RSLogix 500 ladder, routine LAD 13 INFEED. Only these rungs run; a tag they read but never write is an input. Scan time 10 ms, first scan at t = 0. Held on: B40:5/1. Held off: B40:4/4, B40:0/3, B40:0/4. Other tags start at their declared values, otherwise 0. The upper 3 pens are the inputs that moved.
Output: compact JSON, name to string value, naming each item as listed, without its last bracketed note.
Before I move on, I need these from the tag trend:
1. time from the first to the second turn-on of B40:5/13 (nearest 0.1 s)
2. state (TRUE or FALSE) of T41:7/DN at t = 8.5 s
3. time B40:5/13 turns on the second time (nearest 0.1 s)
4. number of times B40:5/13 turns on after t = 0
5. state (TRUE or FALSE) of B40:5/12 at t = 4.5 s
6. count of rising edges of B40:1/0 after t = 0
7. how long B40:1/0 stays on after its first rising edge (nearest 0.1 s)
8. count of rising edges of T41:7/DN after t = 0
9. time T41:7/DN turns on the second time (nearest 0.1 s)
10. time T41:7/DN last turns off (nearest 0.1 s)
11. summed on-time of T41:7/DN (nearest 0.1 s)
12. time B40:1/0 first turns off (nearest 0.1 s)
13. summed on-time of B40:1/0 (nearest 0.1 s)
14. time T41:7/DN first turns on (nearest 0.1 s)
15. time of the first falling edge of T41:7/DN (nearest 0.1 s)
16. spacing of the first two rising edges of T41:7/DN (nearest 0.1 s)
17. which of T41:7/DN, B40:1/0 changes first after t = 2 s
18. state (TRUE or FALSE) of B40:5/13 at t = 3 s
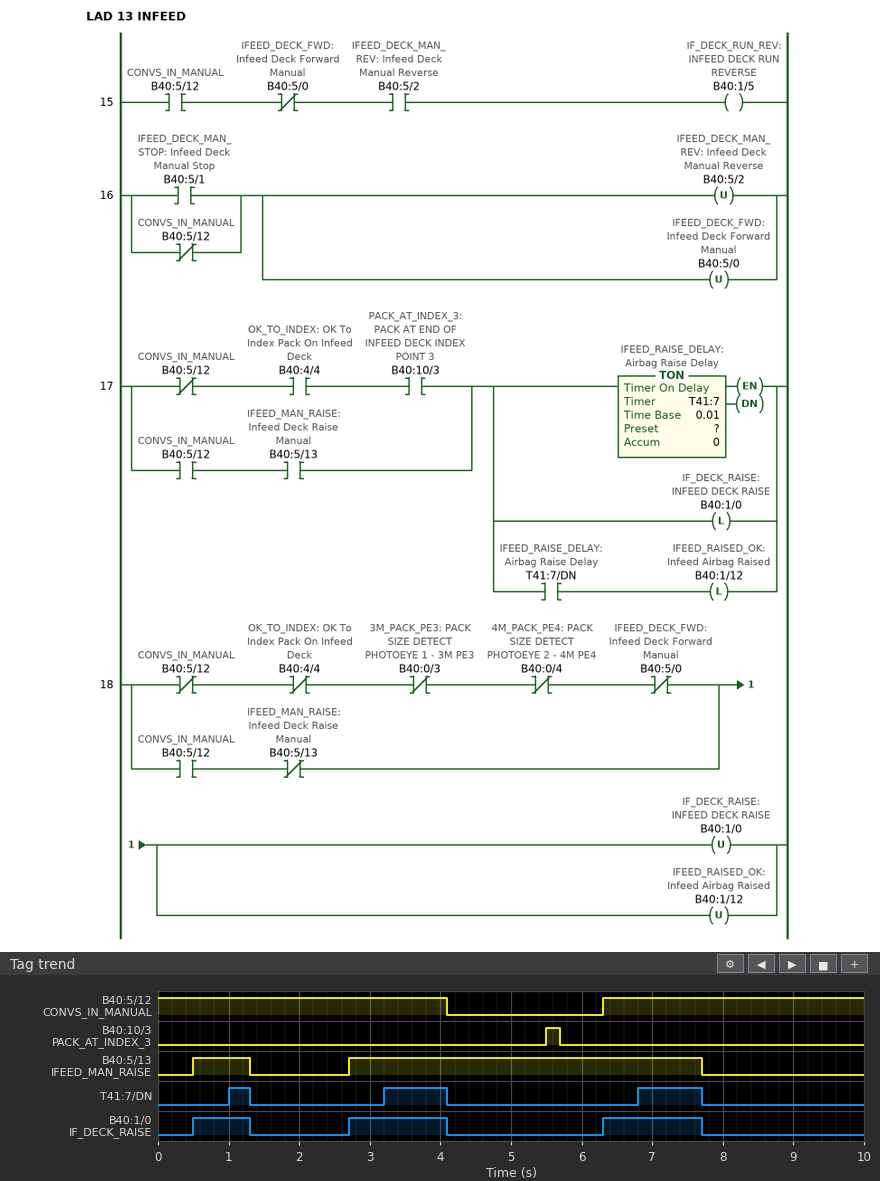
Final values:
{"time from the first to the second turn-on of B40:5/13": "2.2 s", "state (TRUE or FALSE) of T41:7/DN at t = 8.5 s": "FALSE", "time B40:5/13 turns on the second time": "2.7 s", "number of times B40:5/13 turns on after t = 0": "2", "state (TRUE or FALSE) of B40:5/12 at t = 4.5 s": "FALSE", "count of rising edges of B40:1/0 after t = 0": "3", "how long B40:1/0 stays on after its first rising edge": "0.8 s", "count of rising edges of T41:7/DN after t = 0": "3", "time T41:7/DN turns on the second time": "3.2 s", "time T41:7/DN last turns off": "7.7 s", "summed on-time of T41:7/DN": "2.1 s", "time B40:1/0 first turns off": "1.3 s", "summed on-time of B40:1/0": "3.6 s", "time T41:7/DN first turns on": "1.0 s", "time of the first falling edge of T41:7/DN": "1.3 s", "spacing of the first two rising edges of T41:7/DN": "2.2 s", "which of T41:7/DN, B40:1/0 changes first after t = 2 s": "B40:1/0", "state (TRUE or FALSE) of B40:5/13 at t = 3 s": "TRUE"}
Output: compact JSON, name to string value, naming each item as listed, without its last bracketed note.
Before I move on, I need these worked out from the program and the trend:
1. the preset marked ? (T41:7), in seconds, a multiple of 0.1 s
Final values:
{"the preset marked ? (T41:7), in seconds, a multiple of 0.1 s": "0.5 s"}
